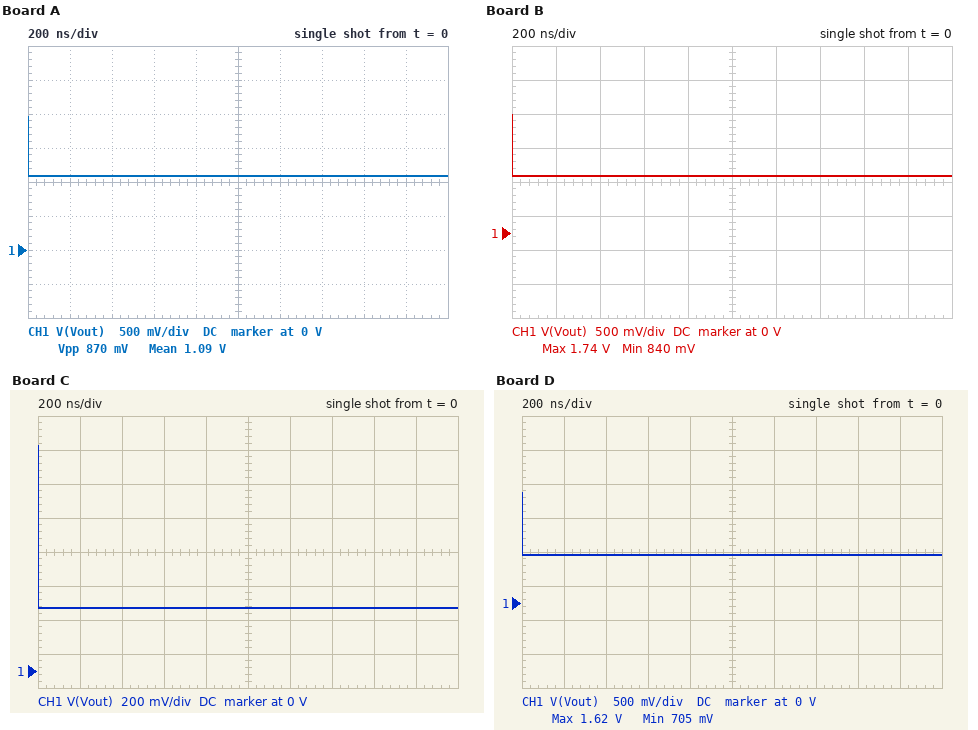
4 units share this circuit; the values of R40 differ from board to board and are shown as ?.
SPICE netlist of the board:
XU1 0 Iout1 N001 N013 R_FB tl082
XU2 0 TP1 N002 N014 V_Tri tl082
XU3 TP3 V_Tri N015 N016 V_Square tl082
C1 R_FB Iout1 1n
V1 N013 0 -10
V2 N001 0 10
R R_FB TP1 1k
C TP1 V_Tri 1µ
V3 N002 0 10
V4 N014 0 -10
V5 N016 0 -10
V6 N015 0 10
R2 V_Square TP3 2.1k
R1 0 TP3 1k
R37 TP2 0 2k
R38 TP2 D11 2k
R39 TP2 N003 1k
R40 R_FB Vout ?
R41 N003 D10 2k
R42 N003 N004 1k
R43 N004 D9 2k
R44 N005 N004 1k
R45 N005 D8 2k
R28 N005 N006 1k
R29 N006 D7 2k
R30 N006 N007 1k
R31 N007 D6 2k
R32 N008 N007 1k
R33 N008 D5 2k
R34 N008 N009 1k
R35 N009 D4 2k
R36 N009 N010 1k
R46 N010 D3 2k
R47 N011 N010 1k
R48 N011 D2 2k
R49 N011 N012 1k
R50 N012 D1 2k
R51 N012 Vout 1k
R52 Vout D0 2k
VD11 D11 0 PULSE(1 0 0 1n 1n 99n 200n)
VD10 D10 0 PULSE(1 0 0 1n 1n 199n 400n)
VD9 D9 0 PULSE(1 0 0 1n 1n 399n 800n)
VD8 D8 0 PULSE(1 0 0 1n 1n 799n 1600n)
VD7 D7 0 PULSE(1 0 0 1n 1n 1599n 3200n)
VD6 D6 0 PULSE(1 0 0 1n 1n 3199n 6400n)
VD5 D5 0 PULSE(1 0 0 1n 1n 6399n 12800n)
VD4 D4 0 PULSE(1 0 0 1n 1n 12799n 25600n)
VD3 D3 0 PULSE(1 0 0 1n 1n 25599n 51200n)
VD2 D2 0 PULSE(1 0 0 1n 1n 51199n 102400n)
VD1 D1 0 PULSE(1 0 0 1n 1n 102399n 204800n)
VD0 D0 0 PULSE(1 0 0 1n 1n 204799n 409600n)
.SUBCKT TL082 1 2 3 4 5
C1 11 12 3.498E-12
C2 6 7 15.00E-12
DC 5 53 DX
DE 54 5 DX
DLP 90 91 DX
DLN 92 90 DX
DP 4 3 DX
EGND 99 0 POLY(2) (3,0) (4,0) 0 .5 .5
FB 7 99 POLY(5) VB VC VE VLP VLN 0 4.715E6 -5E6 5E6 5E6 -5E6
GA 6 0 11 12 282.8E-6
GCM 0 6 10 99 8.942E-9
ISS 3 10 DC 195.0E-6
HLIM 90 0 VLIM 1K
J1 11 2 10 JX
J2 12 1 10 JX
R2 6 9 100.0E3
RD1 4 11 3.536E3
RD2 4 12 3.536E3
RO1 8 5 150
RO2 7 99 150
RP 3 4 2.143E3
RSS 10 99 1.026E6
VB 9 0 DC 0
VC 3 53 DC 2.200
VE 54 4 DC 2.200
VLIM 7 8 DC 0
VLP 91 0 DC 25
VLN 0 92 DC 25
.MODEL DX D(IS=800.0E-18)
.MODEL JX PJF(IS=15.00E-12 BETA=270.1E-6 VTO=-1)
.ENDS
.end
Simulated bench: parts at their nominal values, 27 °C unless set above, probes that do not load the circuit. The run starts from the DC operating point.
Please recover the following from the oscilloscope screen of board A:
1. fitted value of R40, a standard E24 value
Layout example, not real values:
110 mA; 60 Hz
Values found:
6.8 kΩ
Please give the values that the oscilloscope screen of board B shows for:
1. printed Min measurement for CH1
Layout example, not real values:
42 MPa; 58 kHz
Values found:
840 mV
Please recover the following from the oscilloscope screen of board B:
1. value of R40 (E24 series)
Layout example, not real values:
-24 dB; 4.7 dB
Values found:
9.1 kΩ
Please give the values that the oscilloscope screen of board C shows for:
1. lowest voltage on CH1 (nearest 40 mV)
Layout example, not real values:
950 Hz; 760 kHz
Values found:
360 mV
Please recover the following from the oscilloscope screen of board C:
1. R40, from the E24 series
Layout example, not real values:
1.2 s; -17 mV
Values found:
22 kΩ
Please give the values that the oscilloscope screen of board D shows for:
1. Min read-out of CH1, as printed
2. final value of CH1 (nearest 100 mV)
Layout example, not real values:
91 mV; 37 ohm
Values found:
705 mV; 700 mV
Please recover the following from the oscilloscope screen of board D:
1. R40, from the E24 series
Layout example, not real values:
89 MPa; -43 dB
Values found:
11 kΩ
